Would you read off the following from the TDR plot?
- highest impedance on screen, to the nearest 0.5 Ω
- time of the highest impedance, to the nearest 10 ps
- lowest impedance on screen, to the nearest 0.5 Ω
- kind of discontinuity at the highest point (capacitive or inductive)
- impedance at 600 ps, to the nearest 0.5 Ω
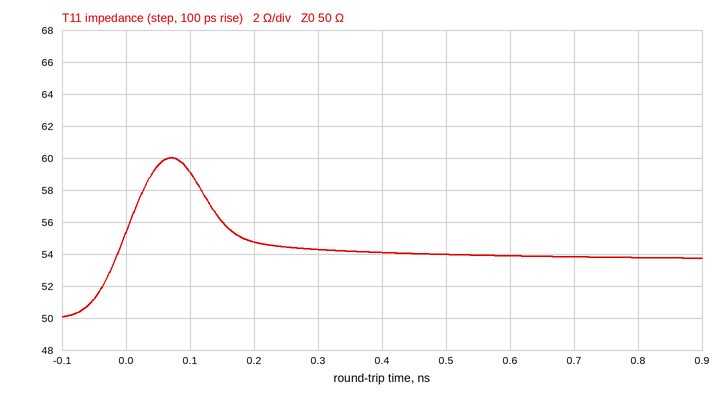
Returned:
60.0 Ω
70 ps
50.0 Ω
inductive
54.0 Ω
